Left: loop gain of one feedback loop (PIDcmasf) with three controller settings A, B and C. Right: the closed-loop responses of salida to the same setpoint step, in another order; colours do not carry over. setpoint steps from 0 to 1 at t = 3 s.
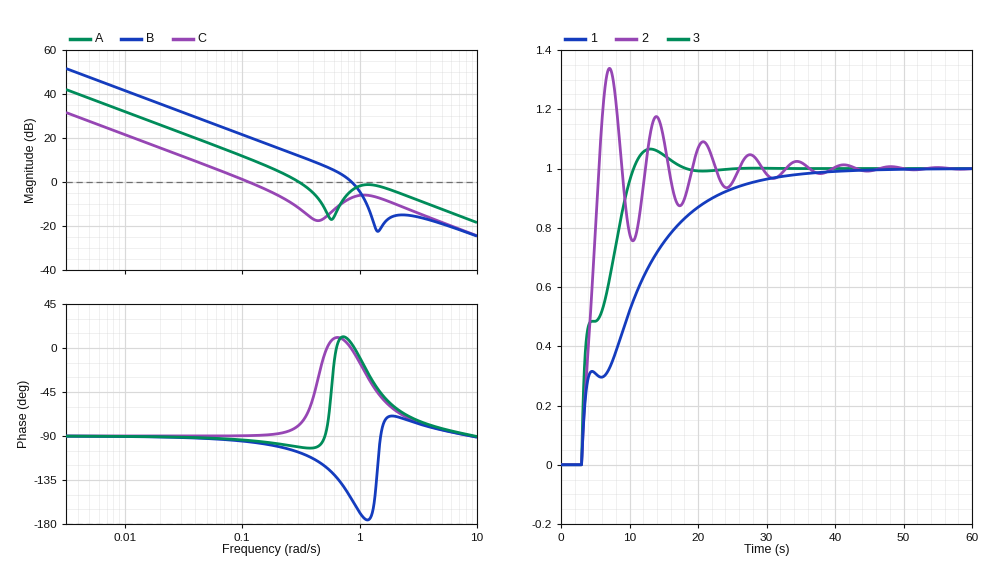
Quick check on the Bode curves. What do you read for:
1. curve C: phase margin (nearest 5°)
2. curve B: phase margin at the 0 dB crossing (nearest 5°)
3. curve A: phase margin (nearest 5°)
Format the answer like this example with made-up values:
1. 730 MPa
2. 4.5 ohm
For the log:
1. 90°
2. 25°
3. 80°
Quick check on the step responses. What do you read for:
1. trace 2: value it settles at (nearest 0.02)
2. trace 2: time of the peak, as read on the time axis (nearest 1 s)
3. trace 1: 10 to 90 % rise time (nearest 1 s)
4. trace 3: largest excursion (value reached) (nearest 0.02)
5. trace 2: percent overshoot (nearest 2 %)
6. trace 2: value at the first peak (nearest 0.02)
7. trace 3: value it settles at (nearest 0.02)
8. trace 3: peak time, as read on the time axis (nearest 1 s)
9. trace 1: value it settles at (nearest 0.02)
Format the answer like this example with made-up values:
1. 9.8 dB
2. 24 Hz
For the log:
1. 1.00
2. 7 s
3. 19 s
4. 1.06
5. 34 %
6. 1.34
7. 1.00
8. 13 s
9. 1.00
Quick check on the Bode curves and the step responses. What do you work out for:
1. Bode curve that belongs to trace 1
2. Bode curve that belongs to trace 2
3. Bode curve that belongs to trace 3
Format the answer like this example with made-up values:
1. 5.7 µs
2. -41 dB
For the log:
1. C
2. B
3. A
